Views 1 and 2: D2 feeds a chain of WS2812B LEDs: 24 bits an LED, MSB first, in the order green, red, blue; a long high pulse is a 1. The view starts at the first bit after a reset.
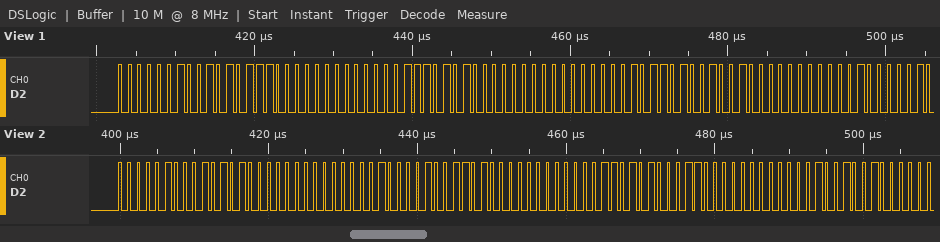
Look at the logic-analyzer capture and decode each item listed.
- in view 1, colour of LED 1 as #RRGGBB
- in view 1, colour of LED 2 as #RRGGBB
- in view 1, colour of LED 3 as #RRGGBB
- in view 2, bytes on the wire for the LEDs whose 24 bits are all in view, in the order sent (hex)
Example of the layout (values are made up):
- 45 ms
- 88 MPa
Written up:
- #570200
- #500700
- #490B00
- 04 54 00 08 4D 00 0D 46 00
